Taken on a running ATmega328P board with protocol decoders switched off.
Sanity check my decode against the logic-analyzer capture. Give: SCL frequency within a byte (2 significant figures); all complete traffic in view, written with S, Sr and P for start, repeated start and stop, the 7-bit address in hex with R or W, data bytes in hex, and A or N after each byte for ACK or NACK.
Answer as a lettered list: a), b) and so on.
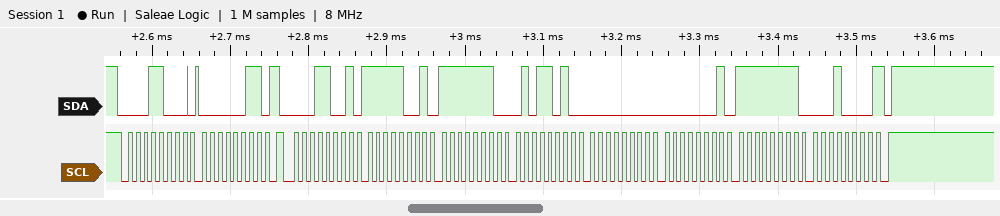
a) 100 kHz
b) S 0CW A 03 A Sr 0CR A F9 A FE A 5A A 00 A 01 A FF A 10 N P
